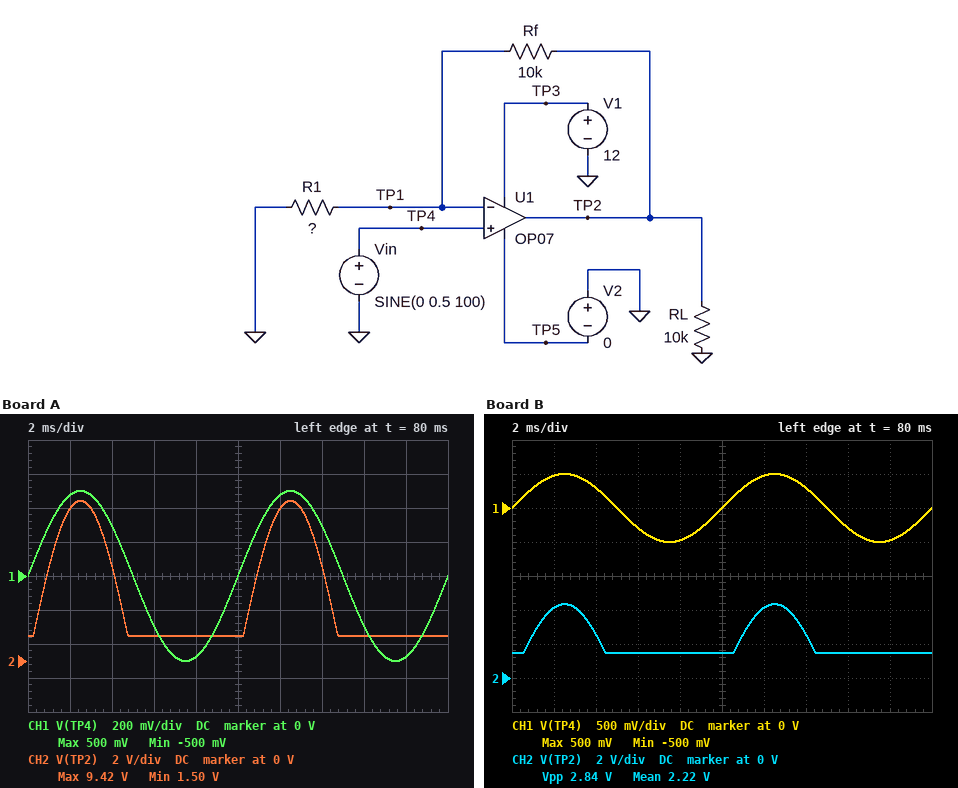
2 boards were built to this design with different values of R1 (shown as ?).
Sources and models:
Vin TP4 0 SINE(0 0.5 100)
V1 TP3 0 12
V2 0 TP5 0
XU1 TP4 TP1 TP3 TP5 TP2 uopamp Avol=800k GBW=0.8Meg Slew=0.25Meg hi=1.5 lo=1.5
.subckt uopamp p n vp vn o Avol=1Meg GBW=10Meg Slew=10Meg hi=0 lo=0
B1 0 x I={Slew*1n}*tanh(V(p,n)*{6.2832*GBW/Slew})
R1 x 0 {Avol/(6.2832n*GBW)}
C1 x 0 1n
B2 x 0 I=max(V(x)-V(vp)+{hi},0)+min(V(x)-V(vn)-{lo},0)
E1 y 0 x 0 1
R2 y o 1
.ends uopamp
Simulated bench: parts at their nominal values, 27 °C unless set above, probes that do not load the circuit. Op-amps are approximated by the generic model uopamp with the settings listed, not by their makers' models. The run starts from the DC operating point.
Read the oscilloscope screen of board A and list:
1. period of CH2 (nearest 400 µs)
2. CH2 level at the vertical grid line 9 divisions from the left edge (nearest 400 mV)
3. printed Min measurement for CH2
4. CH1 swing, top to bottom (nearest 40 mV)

10.0 ms
1.6 V
1.50 V
1.00 V
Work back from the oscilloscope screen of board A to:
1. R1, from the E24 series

560 Ω
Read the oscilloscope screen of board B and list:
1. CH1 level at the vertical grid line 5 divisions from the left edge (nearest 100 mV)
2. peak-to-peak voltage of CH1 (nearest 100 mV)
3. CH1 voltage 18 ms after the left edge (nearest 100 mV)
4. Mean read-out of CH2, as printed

0 V
1.0 V
-500 mV
2.22 V
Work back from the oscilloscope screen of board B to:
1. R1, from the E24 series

1.3 kΩ
